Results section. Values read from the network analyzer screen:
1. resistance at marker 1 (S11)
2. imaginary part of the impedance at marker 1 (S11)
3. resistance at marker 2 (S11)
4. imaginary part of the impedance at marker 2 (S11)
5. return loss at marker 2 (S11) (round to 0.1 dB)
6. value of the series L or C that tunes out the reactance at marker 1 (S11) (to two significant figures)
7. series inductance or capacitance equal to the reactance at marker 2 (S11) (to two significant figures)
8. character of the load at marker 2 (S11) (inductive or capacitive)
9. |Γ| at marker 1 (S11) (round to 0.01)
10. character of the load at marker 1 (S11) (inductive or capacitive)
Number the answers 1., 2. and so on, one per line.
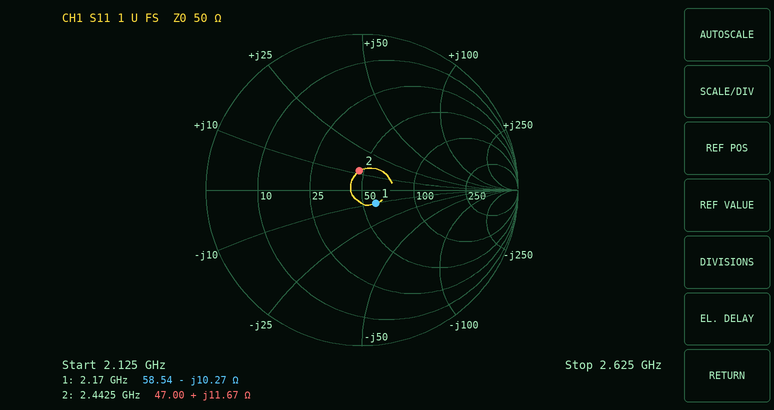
1. 58.54 Ω
2. -10.27 Ω
3. 47.00 Ω
4. +11.67 Ω
5. 18.2 dB
6. 750 pH
7. 760 pH
8. inductive
9. 0.12
10. capacitive
